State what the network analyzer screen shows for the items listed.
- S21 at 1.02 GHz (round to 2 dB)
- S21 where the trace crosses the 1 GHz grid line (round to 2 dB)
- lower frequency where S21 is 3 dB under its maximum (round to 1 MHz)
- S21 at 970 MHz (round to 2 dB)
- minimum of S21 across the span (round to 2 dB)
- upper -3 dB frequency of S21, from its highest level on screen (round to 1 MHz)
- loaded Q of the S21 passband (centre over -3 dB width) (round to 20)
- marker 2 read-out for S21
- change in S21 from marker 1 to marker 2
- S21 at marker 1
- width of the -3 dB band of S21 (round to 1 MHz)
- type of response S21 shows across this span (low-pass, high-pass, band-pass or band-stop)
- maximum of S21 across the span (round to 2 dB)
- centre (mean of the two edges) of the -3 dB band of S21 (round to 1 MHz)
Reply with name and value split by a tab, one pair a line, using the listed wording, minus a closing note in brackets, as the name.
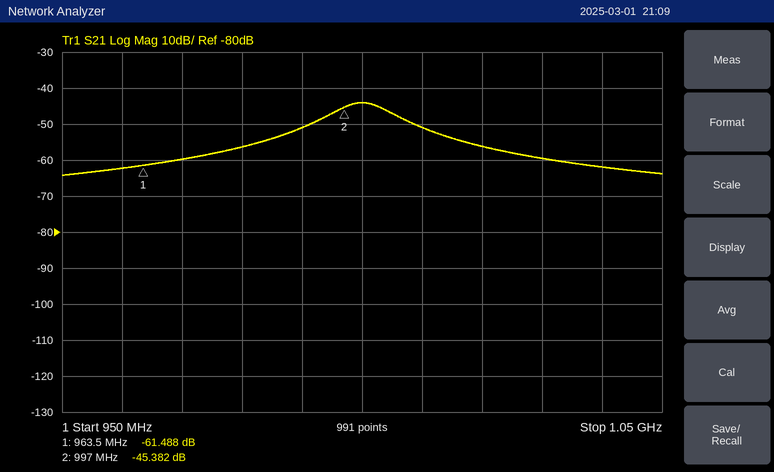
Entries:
S21 at 1.02 GHz	-56 dB
S21 where the trace crosses the 1 GHz grid line	-44 dB
lower frequency where S21 is 3 dB under its maximum	995 MHz
S21 at 970 MHz	-60 dB
minimum of S21 across the span	-64 dB
upper -3 dB frequency of S21, from its highest level on screen	1.005 GHz
loaded Q of the S21 passband (centre over -3 dB width)	100
marker 2 read-out for S21	-45.382 dB
change in S21 from marker 1 to marker 2	16.106 dB
S21 at marker 1	-61.488 dB
width of the -3 dB band of S21	10 MHz
type of response S21 shows across this span	band-pass
maximum of S21 across the span	-44 dB
centre (mean of the two edges) of the -3 dB band of S21	1.000 GHz
